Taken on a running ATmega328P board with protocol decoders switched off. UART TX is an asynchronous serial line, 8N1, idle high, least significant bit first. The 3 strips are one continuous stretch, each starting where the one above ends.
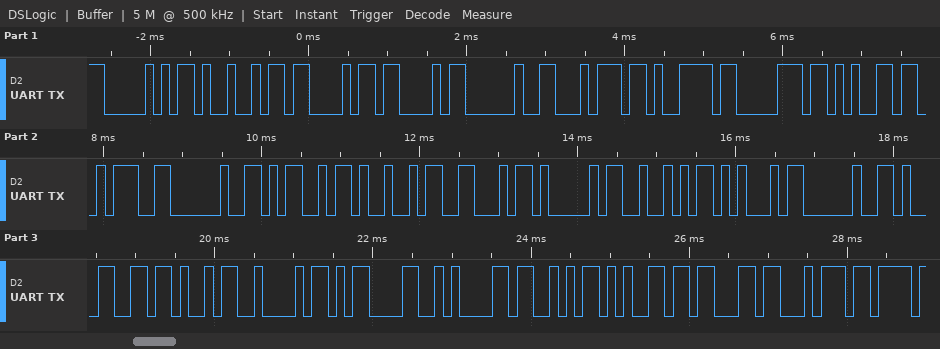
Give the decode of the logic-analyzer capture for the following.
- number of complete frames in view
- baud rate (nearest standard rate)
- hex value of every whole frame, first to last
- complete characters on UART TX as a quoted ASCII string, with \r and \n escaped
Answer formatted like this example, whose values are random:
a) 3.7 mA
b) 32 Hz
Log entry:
a) 27
b) 9600 baud
c) 50 49 43 43 20 74 79 70 65 3A 20 4D 49 46 41 52 45 20 31 4B 42 0D 0A 53 65 63 74
d) "PICC type: MIFARE 1KB\r\nSect"
